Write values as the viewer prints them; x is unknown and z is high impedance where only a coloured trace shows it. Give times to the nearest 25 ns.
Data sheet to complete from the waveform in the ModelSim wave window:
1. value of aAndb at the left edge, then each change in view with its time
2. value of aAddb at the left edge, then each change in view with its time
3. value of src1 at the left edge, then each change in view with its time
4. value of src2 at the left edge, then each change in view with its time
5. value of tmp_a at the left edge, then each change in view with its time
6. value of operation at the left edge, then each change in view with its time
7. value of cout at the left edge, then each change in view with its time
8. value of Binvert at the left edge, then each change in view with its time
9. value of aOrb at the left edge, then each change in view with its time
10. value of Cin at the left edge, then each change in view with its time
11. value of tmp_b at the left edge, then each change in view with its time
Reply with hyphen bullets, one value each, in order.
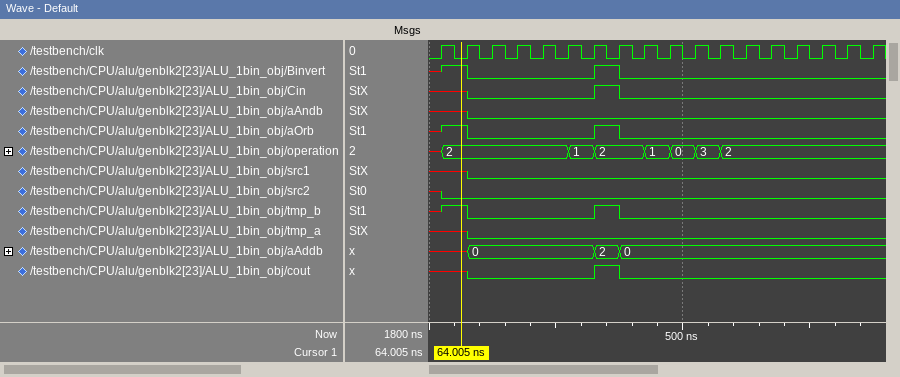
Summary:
- x, 0 at 75 ns
- x, 0 at 75 ns, 2 at 325 ns, 0 at 375 ns
- x, 0 at 75 ns
- x, 0 at 25 ns
- x, 0 at 75 ns
- x, 2 at 25 ns, 1 at 275 ns, 2 at 325 ns, 1 at 425 ns, 0 at 475 ns, 3 at 525 ns, 2 at 575 ns
- x, 0 at 75 ns, 1 at 325 ns, 0 at 375 ns
- x, 1 at 25 ns, 0 at 75 ns, 1 at 325 ns, 0 at 375 ns
- x, 1 at 25 ns, 0 at 75 ns, 1 at 325 ns, 0 at 375 ns
- x, 0 at 75 ns, 1 at 325 ns, 0 at 375 ns
- x, 1 at 25 ns, 0 at 75 ns, 1 at 325 ns, 0 at 375 ns
